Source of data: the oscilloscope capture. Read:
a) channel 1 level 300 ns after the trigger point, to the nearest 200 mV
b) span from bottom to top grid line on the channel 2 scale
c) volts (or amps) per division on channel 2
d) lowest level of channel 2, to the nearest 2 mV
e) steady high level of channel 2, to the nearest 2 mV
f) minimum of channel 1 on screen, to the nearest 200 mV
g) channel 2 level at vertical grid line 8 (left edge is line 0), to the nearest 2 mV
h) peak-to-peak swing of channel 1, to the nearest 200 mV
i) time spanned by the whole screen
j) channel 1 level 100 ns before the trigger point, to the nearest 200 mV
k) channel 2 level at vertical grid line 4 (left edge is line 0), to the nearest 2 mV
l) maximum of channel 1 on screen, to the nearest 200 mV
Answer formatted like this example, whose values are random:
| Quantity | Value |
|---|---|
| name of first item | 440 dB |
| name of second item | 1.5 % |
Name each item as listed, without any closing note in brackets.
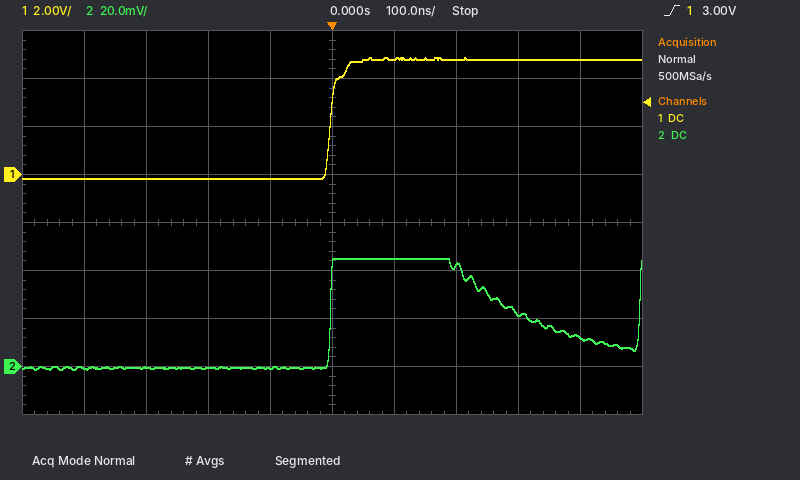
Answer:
| Quantity | Value |
|---|---|
| channel 1 level 300 ns after the trigger point, to the nearest 200 mV | 4.8 V |
| span from bottom to top grid line on the channel 2 scale | 160 mV |
| volts (or amps) per division on channel 2 | 20 mV |
| lowest level of channel 2, to the nearest 2 mV | -2 mV |
| steady high level of channel 2, to the nearest 2 mV | 44 mV |
| minimum of channel 1 on screen, to the nearest 200 mV | -200 mV |
| channel 2 level at vertical grid line 8 (left edge is line 0), to the nearest 2 mV | 22 mV |
| peak-to-peak swing of channel 1, to the nearest 200 mV | 5.0 V |
| time spanned by the whole screen | 1 µs |
| channel 1 level 100 ns before the trigger point, to the nearest 200 mV | -200 mV |
| channel 2 level at vertical grid line 4 (left edge is line 0), to the nearest 2 mV | 0 mV |
| maximum of channel 1 on screen, to the nearest 200 mV | 4.8 V |
